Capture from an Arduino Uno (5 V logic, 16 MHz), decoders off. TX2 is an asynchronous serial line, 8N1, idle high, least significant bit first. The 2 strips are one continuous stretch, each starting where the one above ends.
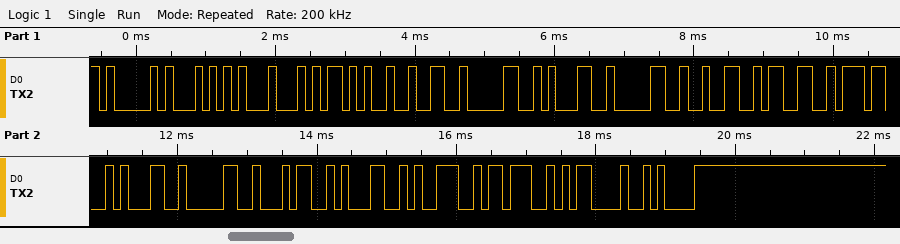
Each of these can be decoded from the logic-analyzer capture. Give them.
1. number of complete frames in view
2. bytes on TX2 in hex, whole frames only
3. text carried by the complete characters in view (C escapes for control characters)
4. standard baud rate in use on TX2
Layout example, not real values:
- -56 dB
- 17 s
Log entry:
- 19
- 41 54 44 2B 32 30 31 30 32 33 37 31 30 34 31 39 3B 0D 0A
- "ATD+201023710419;\r\n"
- 9600 baud
